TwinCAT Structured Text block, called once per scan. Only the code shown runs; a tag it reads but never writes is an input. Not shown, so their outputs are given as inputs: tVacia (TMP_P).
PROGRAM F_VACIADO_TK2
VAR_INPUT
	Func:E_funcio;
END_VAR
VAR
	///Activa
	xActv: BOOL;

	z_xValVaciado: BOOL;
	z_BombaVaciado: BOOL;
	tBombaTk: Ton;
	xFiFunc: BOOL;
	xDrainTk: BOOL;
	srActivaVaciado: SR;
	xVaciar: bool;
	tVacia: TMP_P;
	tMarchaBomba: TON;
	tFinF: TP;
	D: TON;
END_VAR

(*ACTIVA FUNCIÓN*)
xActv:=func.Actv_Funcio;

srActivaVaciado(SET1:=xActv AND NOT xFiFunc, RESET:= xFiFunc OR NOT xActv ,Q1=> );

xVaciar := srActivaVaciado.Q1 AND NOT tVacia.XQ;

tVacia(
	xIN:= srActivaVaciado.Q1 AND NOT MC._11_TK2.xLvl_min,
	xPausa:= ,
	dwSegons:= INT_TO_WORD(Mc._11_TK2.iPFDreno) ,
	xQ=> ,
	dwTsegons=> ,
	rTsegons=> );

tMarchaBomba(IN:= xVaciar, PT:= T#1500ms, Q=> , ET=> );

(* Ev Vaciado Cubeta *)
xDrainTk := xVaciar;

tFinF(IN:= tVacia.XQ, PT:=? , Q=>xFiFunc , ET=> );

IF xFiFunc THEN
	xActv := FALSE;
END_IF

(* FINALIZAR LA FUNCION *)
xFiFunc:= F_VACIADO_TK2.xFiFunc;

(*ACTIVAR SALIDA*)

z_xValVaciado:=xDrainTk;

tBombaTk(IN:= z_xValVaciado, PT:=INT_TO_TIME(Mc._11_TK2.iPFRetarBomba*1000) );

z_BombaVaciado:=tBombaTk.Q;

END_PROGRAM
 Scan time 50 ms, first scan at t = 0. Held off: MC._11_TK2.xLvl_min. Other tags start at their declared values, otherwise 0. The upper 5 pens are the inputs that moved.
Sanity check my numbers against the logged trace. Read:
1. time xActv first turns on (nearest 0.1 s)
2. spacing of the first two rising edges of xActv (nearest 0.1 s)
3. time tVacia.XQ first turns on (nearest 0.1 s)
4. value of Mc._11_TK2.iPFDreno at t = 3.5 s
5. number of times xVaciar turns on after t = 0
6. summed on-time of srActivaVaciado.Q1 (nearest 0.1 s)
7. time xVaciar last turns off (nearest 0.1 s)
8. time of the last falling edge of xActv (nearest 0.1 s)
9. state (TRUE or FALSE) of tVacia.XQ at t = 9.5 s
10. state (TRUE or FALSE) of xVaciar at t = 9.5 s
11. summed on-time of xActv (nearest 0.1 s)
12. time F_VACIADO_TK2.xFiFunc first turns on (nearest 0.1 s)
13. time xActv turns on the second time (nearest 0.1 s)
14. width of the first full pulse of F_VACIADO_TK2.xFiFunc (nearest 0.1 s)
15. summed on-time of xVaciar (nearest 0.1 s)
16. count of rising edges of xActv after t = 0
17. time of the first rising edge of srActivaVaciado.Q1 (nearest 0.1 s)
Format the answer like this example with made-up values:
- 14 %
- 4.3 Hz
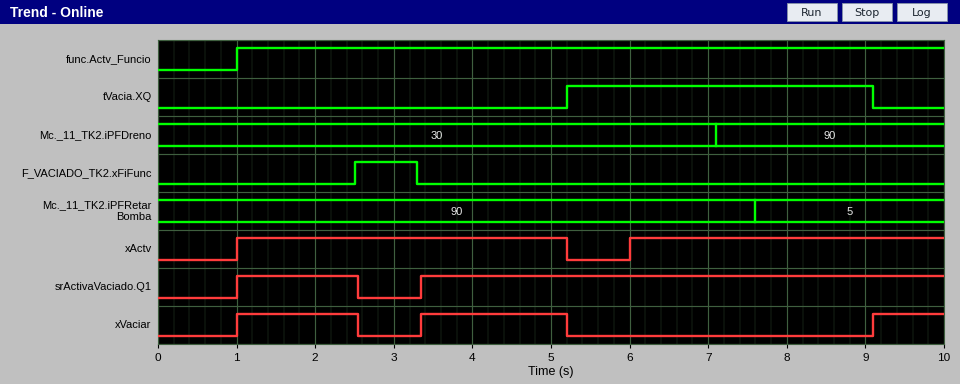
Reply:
- 1.0 s
- 5.0 s
- 5.2 s
- 30
- 3
- 8.2 s
- 5.2 s
- 5.2 s
- FALSE
- TRUE
- 8.2 s
- 2.5 s
- 6.0 s
- 0.8 s
- 4.3 s
- 2
- 1.0 s
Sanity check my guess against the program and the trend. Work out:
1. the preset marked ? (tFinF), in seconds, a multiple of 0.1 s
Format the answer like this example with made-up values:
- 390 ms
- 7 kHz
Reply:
- 0.8 s
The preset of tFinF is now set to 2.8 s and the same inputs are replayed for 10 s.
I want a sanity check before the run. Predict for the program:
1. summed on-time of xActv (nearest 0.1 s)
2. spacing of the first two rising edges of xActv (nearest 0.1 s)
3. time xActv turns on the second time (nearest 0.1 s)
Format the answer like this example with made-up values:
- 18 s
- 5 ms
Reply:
- 6.2 s
- 7.0 s
- 8.0 s
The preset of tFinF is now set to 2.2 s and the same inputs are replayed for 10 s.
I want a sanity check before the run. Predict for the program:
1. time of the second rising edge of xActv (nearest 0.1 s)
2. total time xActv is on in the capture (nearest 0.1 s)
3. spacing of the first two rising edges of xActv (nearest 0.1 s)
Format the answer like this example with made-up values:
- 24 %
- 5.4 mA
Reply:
- 7.4 s
- 6.8 s
- 6.4 s
